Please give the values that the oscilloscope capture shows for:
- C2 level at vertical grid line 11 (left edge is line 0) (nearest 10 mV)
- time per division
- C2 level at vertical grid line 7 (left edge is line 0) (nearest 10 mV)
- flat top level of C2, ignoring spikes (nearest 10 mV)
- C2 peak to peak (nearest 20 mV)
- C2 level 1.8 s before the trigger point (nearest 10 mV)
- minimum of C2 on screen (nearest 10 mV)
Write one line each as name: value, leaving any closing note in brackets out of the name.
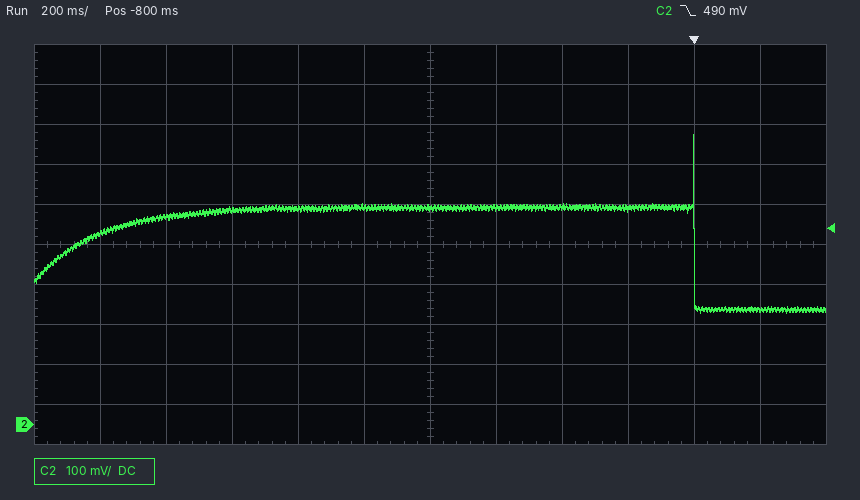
C2 level at vertical grid line 11 (left edge is line 0): 290 mV
time per division: 200 ms
C2 level at vertical grid line 7 (left edge is line 0): 540 mV
flat top level of C2, ignoring spikes: 540 mV
C2 peak to peak: 440 mV
C2 level 1.8 s before the trigger point: 480 mV
minimum of C2 on screen: 280 mV
